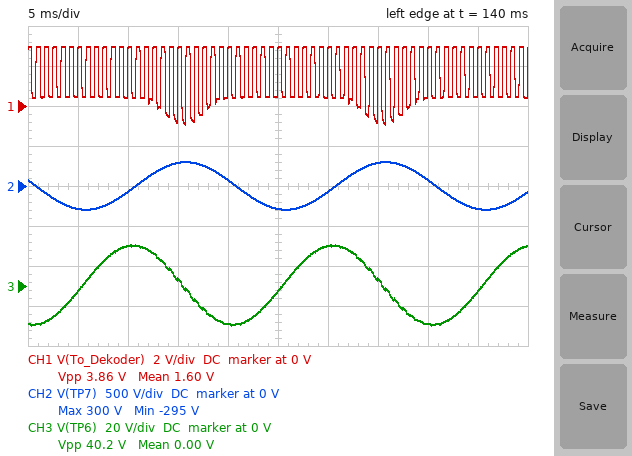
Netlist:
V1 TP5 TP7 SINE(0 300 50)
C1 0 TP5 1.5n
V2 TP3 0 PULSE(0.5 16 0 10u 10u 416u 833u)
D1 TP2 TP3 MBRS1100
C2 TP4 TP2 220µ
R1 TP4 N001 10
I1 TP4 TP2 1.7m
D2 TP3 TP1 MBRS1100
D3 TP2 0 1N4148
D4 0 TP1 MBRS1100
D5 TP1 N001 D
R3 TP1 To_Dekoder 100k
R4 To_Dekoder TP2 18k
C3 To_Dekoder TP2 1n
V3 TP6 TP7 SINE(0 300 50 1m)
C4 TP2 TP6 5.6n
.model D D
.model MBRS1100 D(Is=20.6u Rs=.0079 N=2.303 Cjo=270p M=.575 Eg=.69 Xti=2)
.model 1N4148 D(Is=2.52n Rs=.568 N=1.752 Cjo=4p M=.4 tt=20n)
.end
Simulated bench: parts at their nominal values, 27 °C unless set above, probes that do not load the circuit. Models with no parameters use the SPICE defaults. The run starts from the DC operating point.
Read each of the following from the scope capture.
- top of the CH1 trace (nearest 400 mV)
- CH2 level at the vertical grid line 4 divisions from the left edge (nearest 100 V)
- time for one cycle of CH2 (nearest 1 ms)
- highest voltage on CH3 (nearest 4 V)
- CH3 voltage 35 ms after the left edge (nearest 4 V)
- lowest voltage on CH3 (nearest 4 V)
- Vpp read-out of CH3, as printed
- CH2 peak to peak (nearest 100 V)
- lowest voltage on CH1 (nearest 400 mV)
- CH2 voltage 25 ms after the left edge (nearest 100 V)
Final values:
2.8 V
100 V
20 ms
20 V
4 V
-20 V
40.2 V
600 V
-800 mV
-300 V
